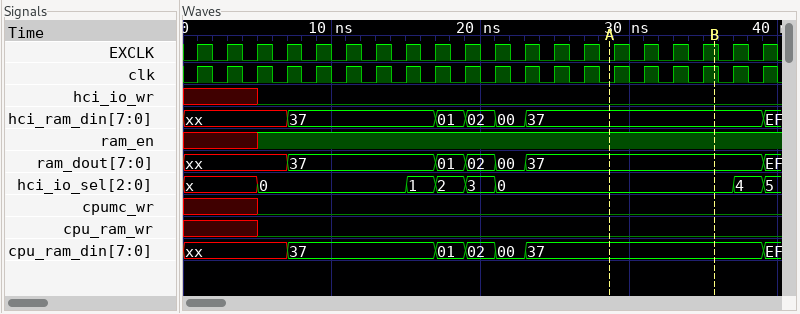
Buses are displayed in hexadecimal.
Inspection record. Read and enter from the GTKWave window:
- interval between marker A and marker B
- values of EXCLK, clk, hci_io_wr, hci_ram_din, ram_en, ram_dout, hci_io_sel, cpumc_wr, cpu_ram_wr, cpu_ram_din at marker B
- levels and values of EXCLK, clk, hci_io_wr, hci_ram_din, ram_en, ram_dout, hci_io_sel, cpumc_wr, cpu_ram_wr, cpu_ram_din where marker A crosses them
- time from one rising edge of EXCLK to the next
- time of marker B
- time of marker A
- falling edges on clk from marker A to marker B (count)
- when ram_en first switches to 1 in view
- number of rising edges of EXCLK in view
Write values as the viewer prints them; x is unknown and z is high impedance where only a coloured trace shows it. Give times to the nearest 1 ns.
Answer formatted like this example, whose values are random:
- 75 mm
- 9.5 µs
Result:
- 7 ns
- EXCLK=1, clk=1, hci_io_wr=0, hci_ram_din=37, ram_en=1, ram_dout=37, hci_io_sel=0, cpumc_wr=0, cpu_ram_wr=0, cpu_ram_din=37
- EXCLK=0, clk=0, hci_io_wr=0, hci_ram_din=37, ram_en=1, ram_dout=37, hci_io_sel=0, cpumc_wr=0, cpu_ram_wr=0, cpu_ram_din=37
- 2 ns
- 36 ns
- 29 ns
- 3
- 5 ns
- 20
